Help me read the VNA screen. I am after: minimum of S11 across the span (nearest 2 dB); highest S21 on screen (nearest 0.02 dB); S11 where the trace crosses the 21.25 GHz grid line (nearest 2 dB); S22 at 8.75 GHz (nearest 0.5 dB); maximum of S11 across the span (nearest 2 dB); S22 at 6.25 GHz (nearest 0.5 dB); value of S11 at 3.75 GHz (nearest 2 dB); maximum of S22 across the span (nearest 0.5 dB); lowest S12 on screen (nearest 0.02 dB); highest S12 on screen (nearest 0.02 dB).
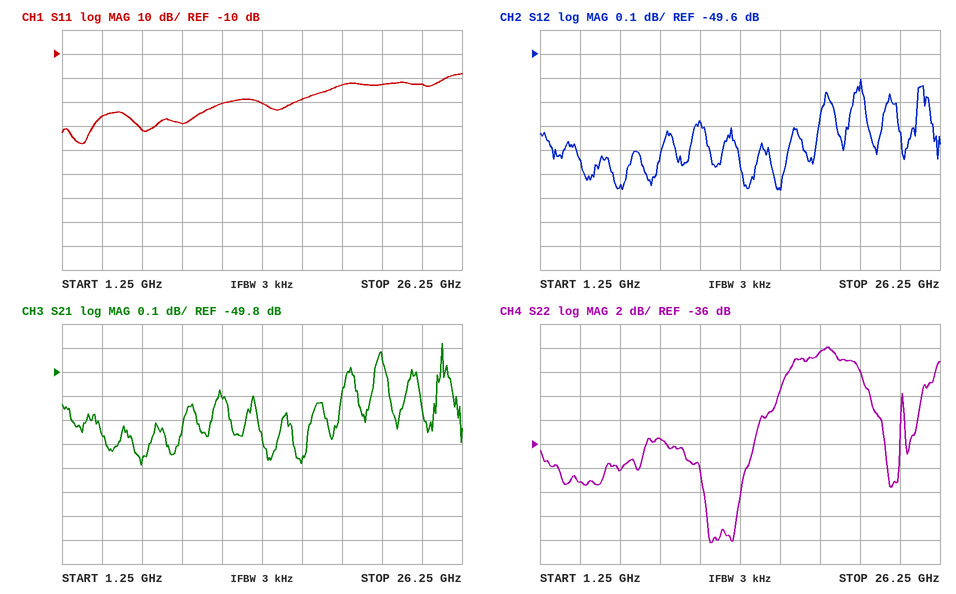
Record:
-48 dB
-49.68 dB
-22 dB
-35.5 dB
-18 dB
-38.0 dB
-36 dB
-28.0 dB
-50.16 dB
-49.70 dB
